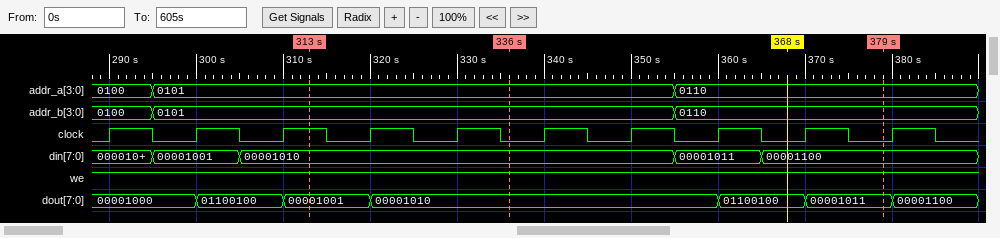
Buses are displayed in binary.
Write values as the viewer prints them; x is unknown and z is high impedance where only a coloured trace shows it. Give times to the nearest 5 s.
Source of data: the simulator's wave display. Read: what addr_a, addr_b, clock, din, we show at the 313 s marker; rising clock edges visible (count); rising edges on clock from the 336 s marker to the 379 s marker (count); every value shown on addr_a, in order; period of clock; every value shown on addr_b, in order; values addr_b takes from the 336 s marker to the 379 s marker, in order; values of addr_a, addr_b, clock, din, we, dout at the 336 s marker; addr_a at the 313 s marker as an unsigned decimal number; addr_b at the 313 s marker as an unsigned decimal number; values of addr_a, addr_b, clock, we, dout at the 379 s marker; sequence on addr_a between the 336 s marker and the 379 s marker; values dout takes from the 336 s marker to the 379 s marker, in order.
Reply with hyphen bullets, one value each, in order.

- addr_a=0101, addr_b=0101, clock=1, din=00001010, we=1
- 10
- 4
- 0100, 0101, 0110
- 10 s
- 0100, 0101, 0110
- 0101, 0110
- addr_a=0101, addr_b=0101, clock=0, din=00001010, we=1, dout=00001010
- 5
- 5
- addr_a=0110, addr_b=0110, clock=0, we=1, dout=00001011
- 0101, 0110
- 00001010, 01100100, 00001011
